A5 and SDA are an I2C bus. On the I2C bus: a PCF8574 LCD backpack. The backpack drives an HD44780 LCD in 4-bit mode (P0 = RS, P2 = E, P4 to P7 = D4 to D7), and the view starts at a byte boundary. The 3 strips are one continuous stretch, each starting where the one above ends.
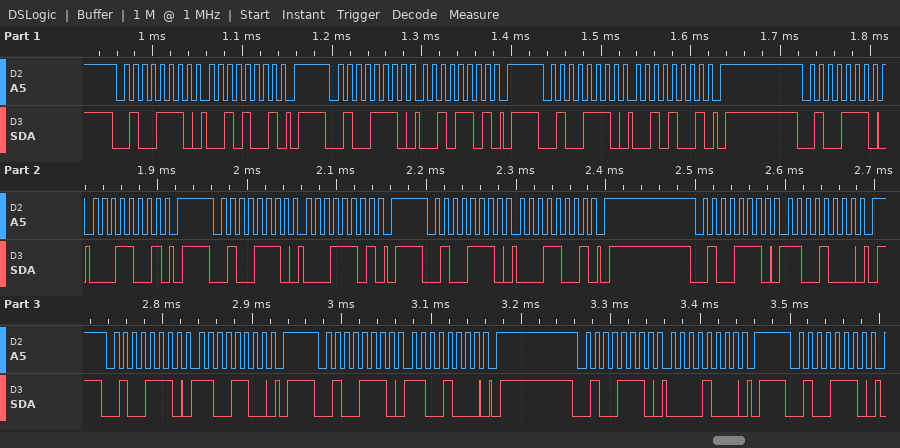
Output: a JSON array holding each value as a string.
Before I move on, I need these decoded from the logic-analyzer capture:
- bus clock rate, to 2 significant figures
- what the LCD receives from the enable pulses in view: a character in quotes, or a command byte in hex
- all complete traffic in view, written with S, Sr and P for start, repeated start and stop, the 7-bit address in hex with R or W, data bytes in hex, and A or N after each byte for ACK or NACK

["100 kHz", "'!'", "S 27W A 29 A P S 27W A 2D A P S 27W A 29 A P S 27W A 19 A P S 27W A 1D A P S 27W A 19 A P S 27W A C8 A P S 27W A CC A P S 27W A C8 A P S 27W A 08 A P S 27W A"]
